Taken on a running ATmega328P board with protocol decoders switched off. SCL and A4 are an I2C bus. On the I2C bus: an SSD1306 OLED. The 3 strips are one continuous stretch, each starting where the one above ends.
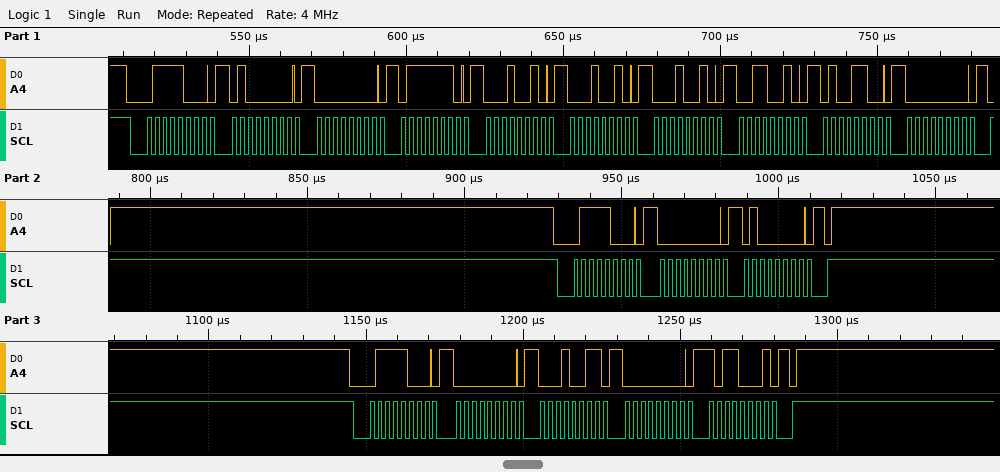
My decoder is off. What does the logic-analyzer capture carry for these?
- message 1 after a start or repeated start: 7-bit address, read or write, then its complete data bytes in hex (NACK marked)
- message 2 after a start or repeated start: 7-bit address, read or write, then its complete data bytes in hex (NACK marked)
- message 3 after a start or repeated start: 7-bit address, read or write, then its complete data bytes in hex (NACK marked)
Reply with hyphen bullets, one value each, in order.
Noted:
- 0x3C write: 40 00 7E 12 12 12 32 4C 00
- 0x3C write: 00 40
- 0x3C write: 00 13 00 B1
